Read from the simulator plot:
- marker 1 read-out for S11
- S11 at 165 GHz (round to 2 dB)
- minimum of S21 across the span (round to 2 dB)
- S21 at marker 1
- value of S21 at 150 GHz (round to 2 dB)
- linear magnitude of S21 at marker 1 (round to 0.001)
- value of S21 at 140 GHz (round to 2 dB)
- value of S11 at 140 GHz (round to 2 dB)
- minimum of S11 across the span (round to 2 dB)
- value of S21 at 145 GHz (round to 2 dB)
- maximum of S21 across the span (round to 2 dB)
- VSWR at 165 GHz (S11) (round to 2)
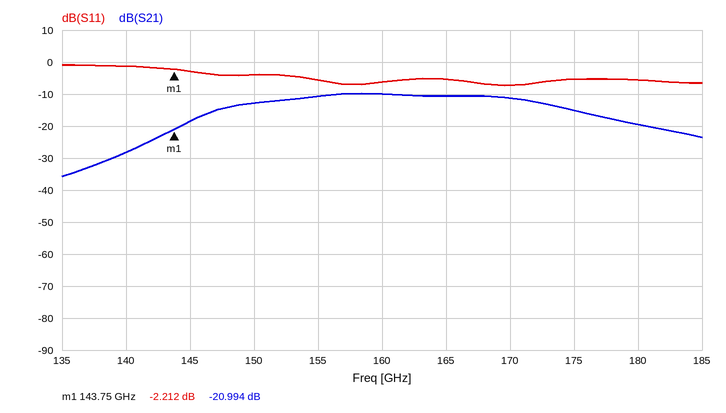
-2.212 dB
-6 dB
-36 dB
-20.994 dB
-12 dB
0.089
-28 dB
-2 dB
-8 dB
-18 dB
-10 dB
4
